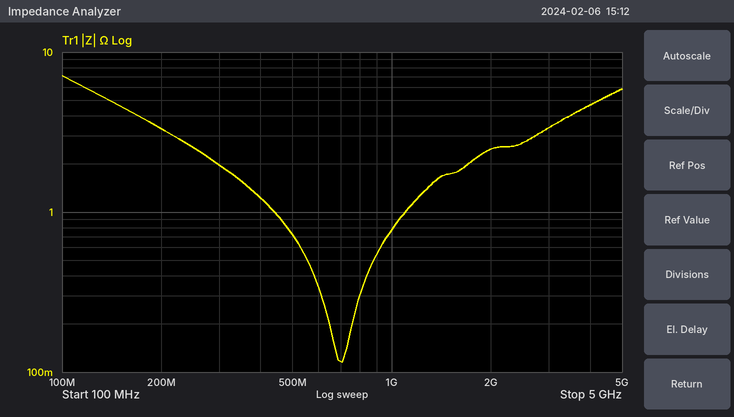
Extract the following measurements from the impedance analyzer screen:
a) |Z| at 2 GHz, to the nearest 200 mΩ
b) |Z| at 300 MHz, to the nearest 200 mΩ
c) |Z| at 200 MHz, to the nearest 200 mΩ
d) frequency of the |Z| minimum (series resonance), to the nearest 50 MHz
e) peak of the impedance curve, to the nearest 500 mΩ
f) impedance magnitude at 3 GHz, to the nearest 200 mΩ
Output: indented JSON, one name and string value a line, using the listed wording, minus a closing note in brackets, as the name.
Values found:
{
  "|Z| at 2 GHz, to the nearest 200 mΩ": "2.4 Ω",
  "|Z| at 300 MHz, to the nearest 200 mΩ": "2.0 Ω",
  "|Z| at 200 MHz, to the nearest 200 mΩ": "3.4 Ω",
  "frequency of the |Z| minimum (series resonance), to the nearest 50 MHz": "700 MHz",
  "peak of the impedance curve, to the nearest 500 mΩ": "7.0 Ω",
  "impedance magnitude at 3 GHz, to the nearest 200 mΩ": "3.4 Ω"
}
